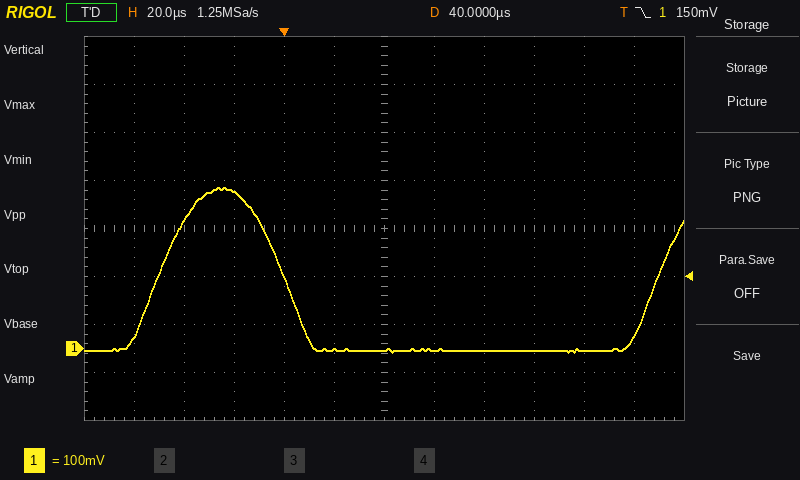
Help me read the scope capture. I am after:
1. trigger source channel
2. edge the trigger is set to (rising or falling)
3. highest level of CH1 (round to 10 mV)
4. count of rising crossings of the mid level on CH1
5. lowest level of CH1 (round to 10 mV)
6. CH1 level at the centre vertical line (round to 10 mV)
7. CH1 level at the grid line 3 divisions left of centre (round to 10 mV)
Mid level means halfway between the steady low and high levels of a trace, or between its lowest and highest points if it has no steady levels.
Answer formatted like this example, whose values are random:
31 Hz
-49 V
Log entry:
CH1
falling
340 mV
2
-10 mV
0 mV
330 mV
